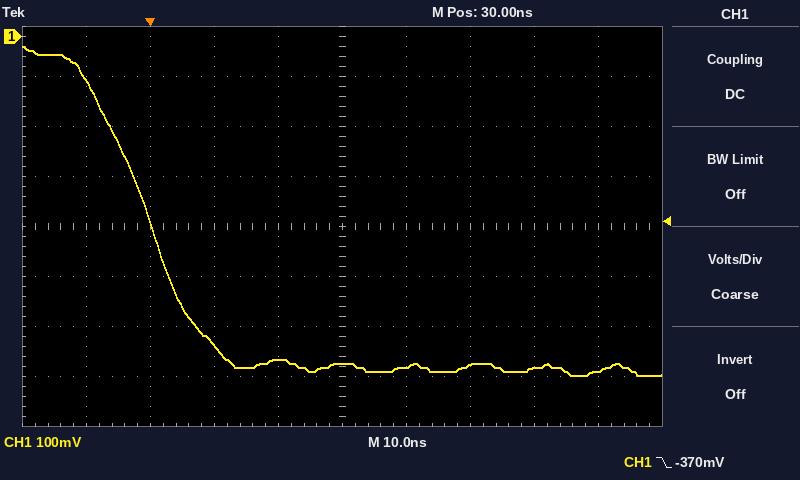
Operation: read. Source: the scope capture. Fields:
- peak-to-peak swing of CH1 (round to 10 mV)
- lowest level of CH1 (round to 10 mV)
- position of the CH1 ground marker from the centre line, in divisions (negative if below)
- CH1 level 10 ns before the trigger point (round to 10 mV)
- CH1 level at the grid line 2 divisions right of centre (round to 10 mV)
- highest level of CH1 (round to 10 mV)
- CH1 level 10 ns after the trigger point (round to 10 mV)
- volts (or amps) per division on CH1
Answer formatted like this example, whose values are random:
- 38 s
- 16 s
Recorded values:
- 660 mV
- -680 mV
- +3.8 div
- -90 mV
- -660 mV
- -20 mV
- -620 mV
- 100 mV
